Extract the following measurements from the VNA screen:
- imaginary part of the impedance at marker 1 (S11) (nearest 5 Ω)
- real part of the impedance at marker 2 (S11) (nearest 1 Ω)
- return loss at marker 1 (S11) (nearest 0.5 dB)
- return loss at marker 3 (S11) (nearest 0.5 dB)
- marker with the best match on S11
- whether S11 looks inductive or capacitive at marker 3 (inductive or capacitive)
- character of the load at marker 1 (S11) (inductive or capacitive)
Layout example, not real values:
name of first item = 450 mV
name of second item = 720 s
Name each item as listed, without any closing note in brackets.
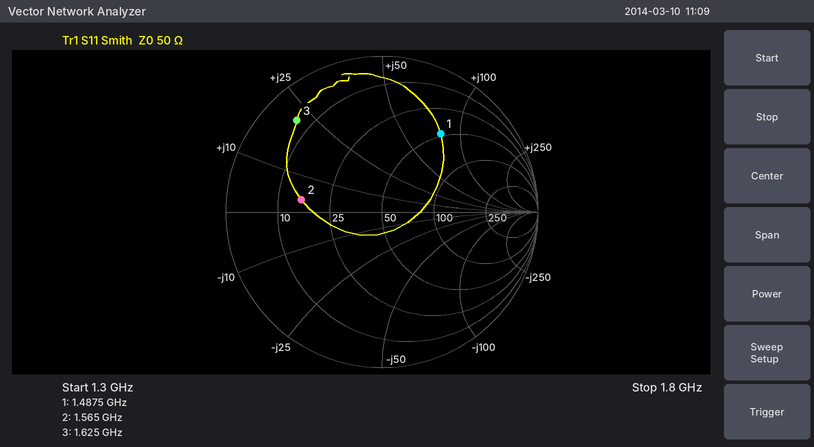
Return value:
imaginary part of the impedance at marker 1 (S11) = +80 Ω
real part of the impedance at marker 2 (S11) = 16 Ω
return loss at marker 1 (S11) = 4.0 dB
return loss at marker 3 (S11) = 2.0 dB
marker with the best match on S11 = marker 2
whether S11 looks inductive or capacitive at marker 3 = inductive
character of the load at marker 1 (S11) = inductive
